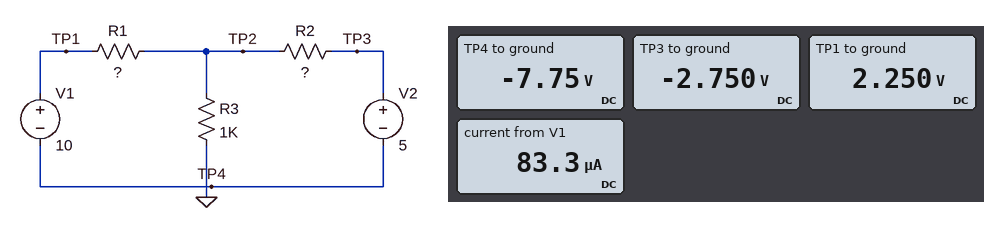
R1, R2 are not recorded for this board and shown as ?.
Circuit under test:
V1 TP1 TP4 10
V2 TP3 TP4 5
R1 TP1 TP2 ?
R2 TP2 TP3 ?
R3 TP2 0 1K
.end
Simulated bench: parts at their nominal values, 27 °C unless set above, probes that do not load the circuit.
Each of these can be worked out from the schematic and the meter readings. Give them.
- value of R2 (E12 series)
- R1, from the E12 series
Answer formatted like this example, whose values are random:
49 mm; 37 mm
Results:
33 kΩ; 27 kΩ
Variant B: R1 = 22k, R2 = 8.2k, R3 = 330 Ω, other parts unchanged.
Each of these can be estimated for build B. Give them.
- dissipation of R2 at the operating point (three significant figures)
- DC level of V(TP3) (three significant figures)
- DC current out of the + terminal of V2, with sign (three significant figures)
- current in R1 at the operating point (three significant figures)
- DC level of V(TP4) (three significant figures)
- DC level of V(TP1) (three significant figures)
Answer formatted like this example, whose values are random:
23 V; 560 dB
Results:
225 µW; -1.36 V; -166 µA; 166 µA; -6.36 V; 3.64 V
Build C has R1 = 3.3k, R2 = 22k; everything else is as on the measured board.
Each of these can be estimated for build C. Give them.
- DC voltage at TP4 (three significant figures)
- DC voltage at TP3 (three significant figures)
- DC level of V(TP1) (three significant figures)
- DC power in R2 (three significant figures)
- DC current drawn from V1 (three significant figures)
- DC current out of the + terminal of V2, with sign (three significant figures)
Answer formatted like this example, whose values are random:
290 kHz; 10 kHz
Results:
-9.35 V; -4.35 V; 652 mV; 859 µW; 198 µA; -198 µA
